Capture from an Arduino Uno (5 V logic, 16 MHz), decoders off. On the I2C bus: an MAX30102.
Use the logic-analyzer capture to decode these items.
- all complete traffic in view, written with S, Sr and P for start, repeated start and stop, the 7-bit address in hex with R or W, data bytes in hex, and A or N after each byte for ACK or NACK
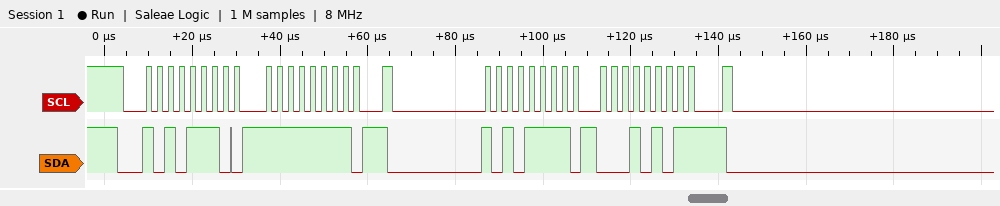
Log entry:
S 57W A FF A Sr 57R A 15 N
